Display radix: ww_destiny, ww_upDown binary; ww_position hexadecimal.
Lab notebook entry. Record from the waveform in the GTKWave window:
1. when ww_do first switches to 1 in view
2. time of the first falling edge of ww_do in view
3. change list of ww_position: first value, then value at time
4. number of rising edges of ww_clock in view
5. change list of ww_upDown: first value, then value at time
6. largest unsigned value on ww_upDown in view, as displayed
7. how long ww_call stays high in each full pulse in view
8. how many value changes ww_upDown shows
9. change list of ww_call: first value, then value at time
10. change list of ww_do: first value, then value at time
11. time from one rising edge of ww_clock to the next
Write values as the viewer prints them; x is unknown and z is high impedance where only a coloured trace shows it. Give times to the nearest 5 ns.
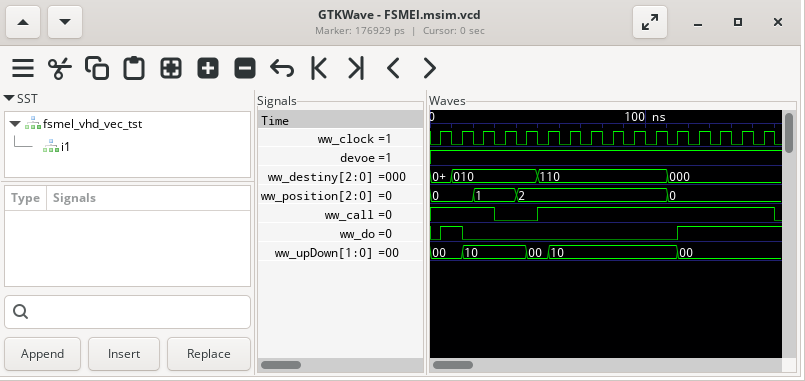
5 ns
15 ns
0, 1 at 20 ns, 2 at 40 ns, 0 at 110 ns
16
00, 10 at 15 ns, 00 at 45 ns, 10 at 55 ns, 00 at 115 ns
10
110 ns
4
1, 0 at 30 ns, 1 at 50 ns, 0 at 160 ns
0, 1 at 5 ns, 0 at 15 ns, 1 at 115 ns
10 ns
